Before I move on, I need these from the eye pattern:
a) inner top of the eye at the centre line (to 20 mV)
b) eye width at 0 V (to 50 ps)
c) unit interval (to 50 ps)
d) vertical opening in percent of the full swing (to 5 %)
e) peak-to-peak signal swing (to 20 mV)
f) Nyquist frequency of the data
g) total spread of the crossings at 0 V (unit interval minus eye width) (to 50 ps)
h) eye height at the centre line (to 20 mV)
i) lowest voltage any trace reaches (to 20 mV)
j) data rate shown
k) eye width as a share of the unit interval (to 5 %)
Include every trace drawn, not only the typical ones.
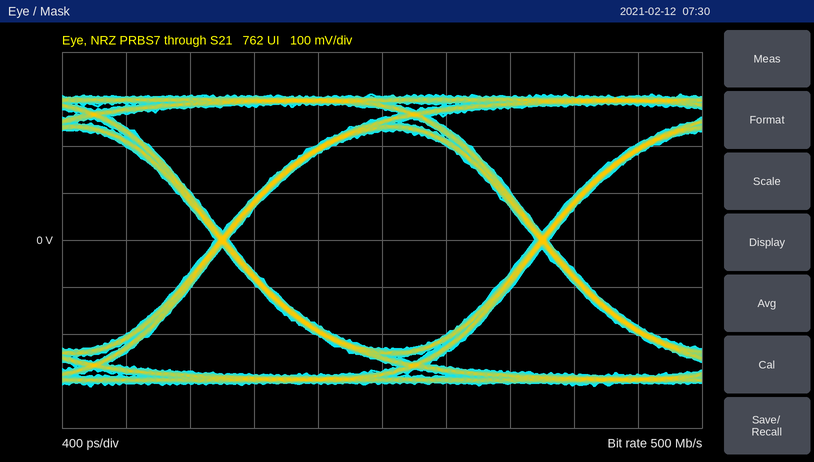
240 mV
1.90 ns
2.00 ns
75 %
620 mV
250 MHz
100 ps
460 mV
-320 mV
500 Mb/s
95 %
